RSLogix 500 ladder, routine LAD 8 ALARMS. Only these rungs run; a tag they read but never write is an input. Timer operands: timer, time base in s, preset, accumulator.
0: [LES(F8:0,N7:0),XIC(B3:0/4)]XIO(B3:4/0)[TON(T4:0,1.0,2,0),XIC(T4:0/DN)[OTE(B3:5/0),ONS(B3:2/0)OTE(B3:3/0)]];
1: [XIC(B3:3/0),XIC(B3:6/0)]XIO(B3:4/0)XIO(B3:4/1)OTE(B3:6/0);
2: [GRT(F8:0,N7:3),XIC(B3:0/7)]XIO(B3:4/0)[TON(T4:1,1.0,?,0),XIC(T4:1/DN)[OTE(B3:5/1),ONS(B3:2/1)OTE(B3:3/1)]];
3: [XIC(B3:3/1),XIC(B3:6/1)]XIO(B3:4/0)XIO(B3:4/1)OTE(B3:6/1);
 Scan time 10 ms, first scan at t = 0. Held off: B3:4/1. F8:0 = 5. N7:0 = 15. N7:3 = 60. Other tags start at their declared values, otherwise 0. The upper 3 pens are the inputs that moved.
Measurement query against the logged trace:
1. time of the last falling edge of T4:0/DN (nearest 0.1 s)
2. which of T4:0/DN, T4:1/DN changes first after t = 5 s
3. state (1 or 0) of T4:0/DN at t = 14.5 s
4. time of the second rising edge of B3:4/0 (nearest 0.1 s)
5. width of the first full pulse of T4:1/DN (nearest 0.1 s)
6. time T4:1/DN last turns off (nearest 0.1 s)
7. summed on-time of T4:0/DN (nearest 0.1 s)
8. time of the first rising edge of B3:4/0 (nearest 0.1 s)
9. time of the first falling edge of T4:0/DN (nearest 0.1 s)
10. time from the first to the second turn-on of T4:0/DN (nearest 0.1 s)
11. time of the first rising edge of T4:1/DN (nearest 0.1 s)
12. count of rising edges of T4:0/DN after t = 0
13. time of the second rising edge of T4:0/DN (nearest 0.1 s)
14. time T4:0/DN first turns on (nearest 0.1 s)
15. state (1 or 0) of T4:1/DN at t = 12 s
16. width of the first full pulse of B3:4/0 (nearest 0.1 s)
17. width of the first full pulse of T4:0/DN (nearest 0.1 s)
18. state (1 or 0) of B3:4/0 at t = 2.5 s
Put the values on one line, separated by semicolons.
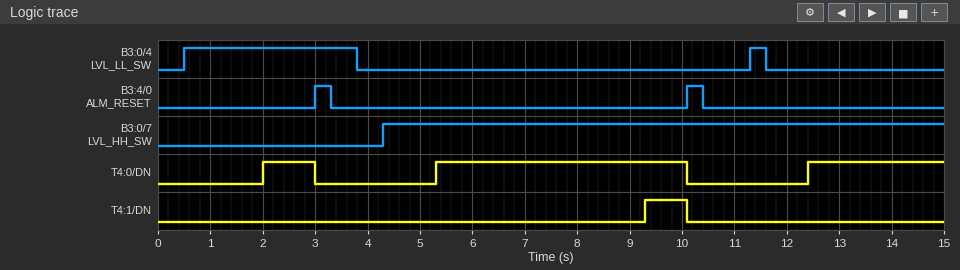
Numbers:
10.1 s; T4:0/DN; 1; 10.1 s; 0.8 s; 10.1 s; 8.4 s; 3.0 s; 3.0 s; 3.3 s; 9.3 s; 3; 5.3 s; 2.0 s; 0; 0.3 s; 1.0 s; 0
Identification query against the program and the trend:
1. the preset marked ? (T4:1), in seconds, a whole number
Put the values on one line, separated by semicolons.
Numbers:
5 s
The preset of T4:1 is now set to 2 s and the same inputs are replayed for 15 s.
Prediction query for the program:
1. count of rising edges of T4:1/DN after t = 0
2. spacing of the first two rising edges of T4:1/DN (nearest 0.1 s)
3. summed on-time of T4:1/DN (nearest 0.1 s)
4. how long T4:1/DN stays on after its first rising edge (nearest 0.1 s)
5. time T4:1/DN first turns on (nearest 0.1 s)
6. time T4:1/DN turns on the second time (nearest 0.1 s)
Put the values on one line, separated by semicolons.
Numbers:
2; 6.1 s; 6.4 s; 3.8 s; 6.3 s; 12.4 s
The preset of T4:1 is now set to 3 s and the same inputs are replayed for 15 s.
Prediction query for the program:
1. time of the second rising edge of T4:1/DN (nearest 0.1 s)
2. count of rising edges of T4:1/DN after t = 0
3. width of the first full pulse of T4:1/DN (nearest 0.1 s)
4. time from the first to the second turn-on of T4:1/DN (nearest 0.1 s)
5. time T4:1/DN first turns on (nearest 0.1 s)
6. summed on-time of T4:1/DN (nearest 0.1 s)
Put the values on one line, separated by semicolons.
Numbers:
13.4 s; 2; 2.8 s; 6.1 s; 7.3 s; 4.4 s
